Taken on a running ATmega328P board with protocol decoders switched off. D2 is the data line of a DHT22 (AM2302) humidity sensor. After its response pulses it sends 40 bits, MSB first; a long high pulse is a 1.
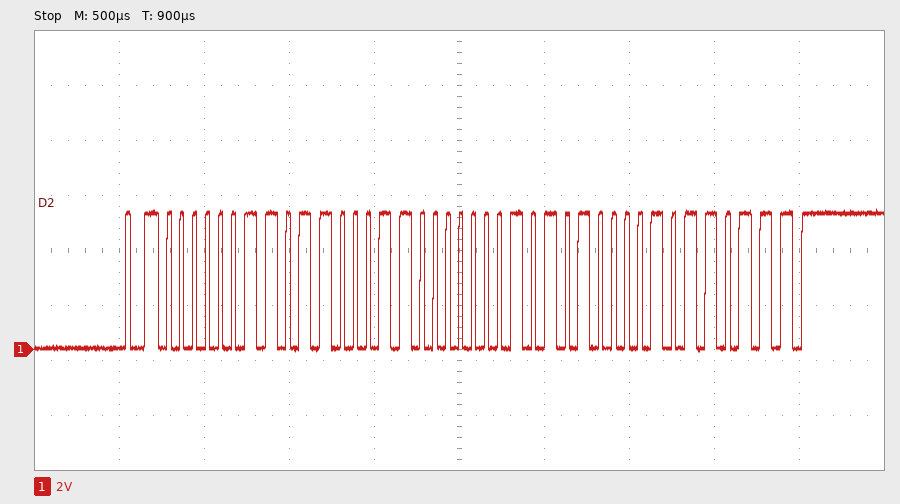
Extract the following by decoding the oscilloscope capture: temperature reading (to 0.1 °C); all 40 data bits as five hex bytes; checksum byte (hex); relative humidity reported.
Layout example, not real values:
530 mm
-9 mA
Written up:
33.6 °C
03 63 01 50 B7
0xB7
86.7 %
